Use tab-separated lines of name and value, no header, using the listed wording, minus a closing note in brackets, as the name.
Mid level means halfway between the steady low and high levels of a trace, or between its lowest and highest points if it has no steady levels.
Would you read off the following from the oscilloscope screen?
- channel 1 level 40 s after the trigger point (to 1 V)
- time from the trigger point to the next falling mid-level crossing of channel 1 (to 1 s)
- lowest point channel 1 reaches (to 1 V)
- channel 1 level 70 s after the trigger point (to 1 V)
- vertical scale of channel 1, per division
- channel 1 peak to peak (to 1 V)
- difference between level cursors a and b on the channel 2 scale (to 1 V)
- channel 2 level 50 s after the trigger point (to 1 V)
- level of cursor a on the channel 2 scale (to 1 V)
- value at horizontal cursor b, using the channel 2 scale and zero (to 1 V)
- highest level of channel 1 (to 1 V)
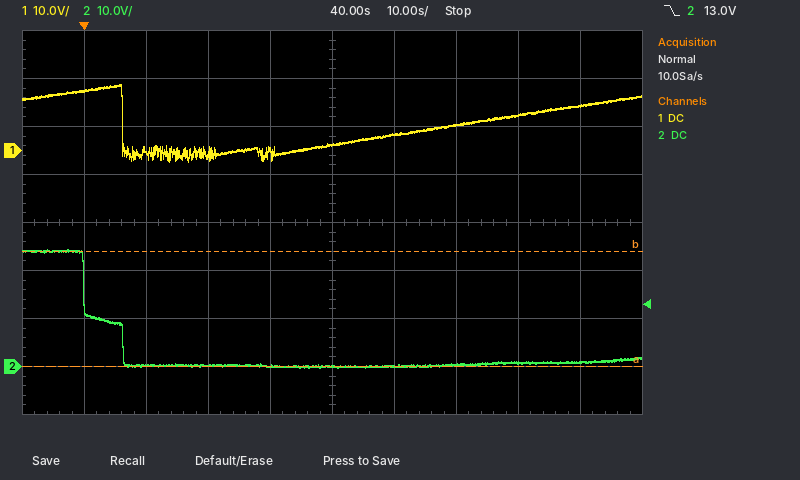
channel 1 level 40 s after the trigger point	1 V
time from the trigger point to the next falling mid-level crossing of channel 1	6 s
lowest point channel 1 reaches	-2 V
channel 1 level 70 s after the trigger point	7 V
vertical scale of channel 1, per division	10 V
channel 1 peak to peak	16 V
difference between level cursors a and b on the channel 2 scale	24 V
channel 2 level 50 s after the trigger point	0 V
level of cursor a on the channel 2 scale	0 V
value at horizontal cursor b, using the channel 2 scale and zero	24 V
highest level of channel 1	14 V
